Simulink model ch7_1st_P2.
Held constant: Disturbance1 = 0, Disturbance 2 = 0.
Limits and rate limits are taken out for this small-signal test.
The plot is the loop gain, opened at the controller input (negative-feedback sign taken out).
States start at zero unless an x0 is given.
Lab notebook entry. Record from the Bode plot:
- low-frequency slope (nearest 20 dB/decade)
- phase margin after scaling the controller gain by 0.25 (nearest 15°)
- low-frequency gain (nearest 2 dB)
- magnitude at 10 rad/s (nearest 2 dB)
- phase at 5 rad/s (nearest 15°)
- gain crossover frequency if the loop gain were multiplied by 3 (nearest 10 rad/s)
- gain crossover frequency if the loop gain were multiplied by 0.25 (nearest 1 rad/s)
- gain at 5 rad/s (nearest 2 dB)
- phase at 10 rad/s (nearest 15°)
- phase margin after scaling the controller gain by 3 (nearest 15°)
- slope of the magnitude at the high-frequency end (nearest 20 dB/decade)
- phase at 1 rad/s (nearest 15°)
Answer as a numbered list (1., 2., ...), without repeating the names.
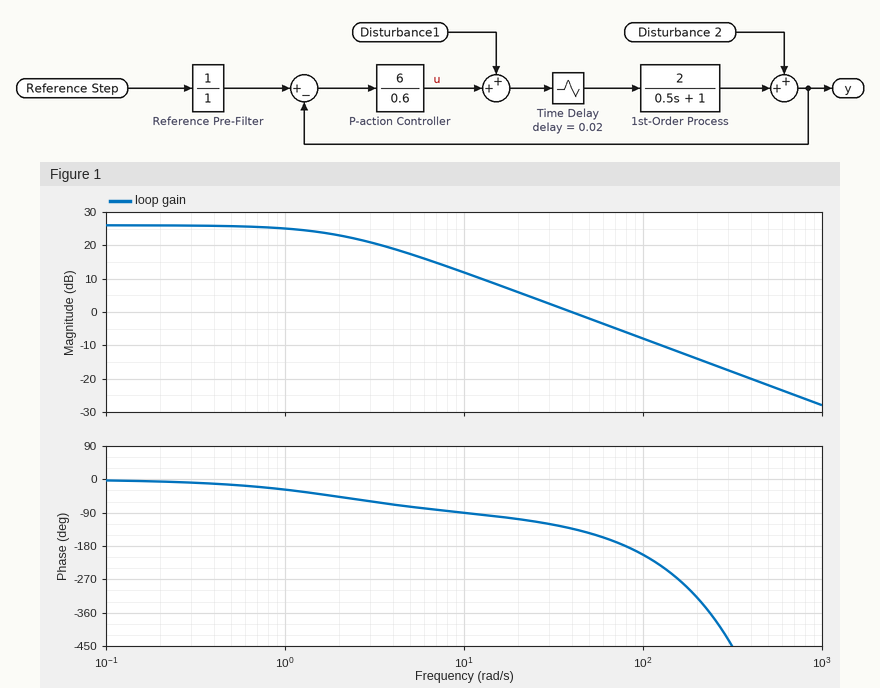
1. 0 dB/decade
2. 90°
3. 26 dB
4. 12 dB
5. -75°
6. 120 rad/s
7. 10 rad/s
8. 18 dB
9. -90°
10. -45°
11. -20 dB/decade
12. -30°
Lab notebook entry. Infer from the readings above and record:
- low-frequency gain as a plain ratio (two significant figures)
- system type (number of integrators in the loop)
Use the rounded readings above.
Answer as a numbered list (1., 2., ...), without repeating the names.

1. 20
2. 0
